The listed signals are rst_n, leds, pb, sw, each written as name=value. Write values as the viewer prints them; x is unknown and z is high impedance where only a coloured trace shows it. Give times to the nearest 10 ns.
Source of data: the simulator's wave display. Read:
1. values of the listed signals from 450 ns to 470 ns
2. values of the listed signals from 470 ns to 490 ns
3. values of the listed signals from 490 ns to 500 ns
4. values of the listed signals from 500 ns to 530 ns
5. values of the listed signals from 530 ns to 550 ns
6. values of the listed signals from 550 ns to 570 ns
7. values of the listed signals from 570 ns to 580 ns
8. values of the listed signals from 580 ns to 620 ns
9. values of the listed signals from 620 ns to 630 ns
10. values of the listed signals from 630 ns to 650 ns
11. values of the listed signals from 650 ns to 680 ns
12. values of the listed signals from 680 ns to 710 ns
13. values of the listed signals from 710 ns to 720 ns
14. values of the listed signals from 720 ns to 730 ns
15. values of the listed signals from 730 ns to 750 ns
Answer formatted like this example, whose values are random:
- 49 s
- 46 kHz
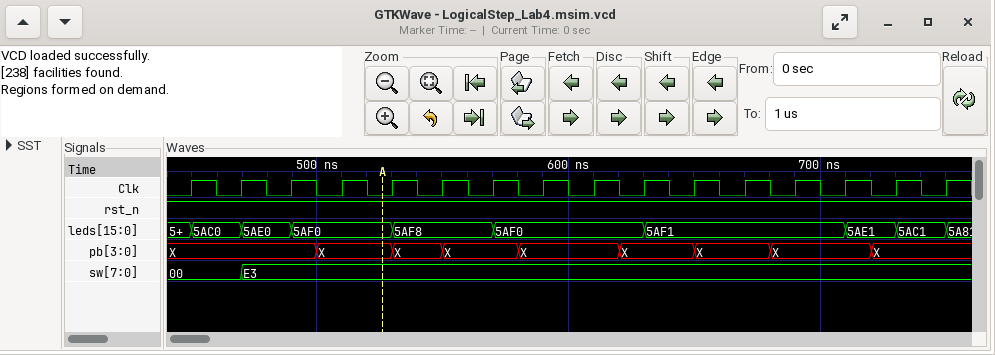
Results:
- rst_n=1, leds=5AC0, pb=X, sw=00
- rst_n=1, leds=5AE0, pb=X, sw=E3
- rst_n=1, leds=5AF0, pb=X, sw=E3
- rst_n=1, leds=5AF0, pb=X, sw=E3
- rst_n=1, leds=5AF8, pb=X, sw=E3
- rst_n=1, leds=5AF8, pb=X, sw=E3
- rst_n=1, leds=5AF0, pb=X, sw=E3
- rst_n=1, leds=5AF0, pb=X, sw=E3
- rst_n=1, leds=5AF0, pb=X, sw=E3
- rst_n=1, leds=5AF1, pb=X, sw=E3
- rst_n=1, leds=5AF1, pb=X, sw=E3
- rst_n=1, leds=5AF1, pb=X, sw=E3
- rst_n=1, leds=5AE1, pb=X, sw=E3
- rst_n=1, leds=5AE1, pb=X, sw=E3
- rst_n=1, leds=5AC1, pb=X, sw=E3
